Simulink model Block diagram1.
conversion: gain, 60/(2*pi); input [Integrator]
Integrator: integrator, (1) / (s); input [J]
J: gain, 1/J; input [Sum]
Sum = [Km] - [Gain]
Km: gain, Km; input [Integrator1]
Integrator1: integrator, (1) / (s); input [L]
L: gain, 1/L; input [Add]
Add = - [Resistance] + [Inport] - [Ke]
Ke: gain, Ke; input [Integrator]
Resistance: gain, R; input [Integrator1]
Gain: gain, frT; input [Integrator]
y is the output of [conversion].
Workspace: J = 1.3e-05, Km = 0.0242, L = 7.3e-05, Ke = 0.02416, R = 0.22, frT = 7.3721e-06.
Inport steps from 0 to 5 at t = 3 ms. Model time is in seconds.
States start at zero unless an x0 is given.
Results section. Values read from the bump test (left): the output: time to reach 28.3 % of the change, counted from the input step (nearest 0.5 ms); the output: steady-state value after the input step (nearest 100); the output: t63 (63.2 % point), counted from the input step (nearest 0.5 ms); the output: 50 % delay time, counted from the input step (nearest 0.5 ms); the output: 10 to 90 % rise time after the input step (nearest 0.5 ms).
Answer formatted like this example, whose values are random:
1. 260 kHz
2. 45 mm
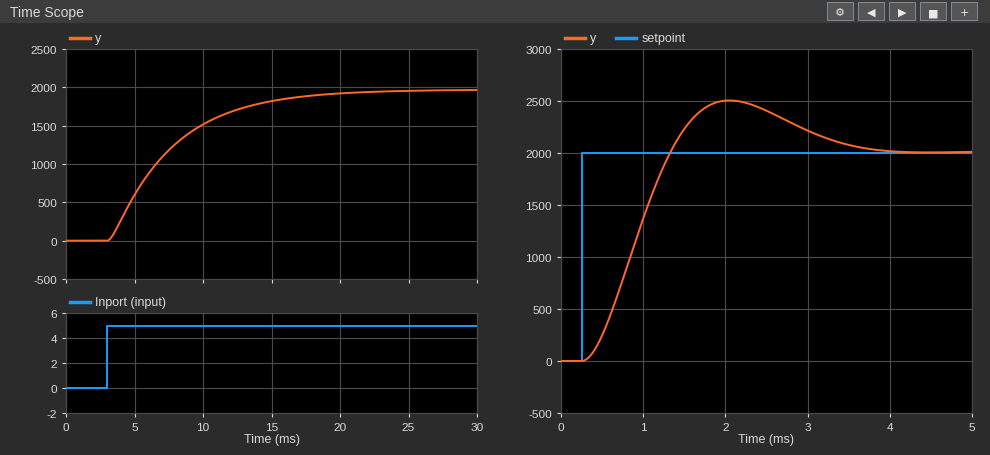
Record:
1. 2.0 ms
2. 2000
3. 5.0 ms
4. 3.5 ms
5. 10.0 ms
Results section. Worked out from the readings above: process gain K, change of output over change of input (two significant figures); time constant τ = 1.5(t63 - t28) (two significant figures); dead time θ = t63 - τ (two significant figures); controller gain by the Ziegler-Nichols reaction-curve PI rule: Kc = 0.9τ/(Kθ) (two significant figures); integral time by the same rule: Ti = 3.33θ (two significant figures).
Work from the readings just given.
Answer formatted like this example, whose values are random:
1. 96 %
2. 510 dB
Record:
1. 400
2. 4.5 ms
3. 0.50 ms
4. 0.020
5. 1.7 ms
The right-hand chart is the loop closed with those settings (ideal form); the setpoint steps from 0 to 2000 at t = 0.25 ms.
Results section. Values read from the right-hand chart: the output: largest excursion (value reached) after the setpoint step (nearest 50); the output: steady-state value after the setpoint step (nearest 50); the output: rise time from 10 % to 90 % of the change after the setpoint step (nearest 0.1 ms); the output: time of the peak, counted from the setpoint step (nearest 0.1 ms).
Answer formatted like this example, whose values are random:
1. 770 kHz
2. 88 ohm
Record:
1. 2500
2. 2000
3. 0.7 ms
4. 1.8 ms
